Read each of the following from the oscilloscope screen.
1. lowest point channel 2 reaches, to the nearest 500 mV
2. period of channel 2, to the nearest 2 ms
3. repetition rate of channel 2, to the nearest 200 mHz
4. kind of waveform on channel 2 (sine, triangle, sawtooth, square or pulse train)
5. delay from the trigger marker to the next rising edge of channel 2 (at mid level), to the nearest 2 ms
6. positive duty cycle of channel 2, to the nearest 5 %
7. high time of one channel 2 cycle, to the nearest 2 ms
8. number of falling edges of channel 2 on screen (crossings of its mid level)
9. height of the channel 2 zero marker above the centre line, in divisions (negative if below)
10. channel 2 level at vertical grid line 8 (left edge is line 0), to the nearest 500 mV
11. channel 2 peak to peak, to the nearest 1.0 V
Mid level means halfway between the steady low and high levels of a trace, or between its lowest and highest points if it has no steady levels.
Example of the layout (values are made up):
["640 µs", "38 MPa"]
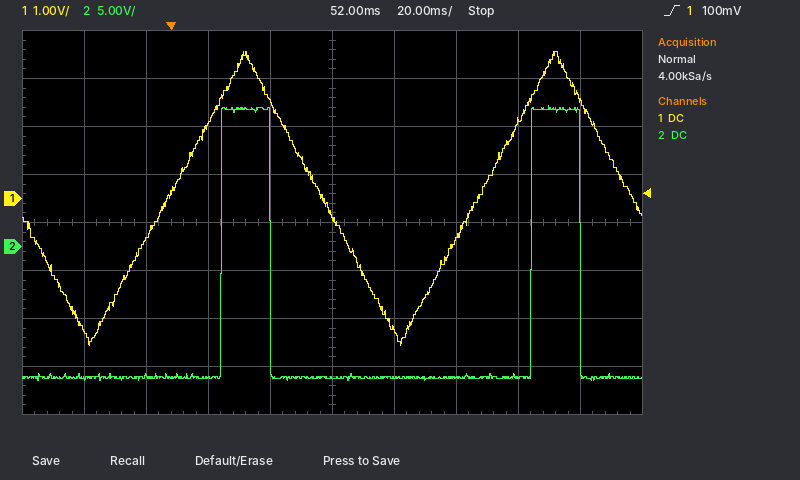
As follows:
["-14.0 V", "100 ms", "10.0 Hz", "pulse train", "16 ms", "15 %", "16 ms", "2", "-0.5 div", "-13.5 V", "29.0 V"]
